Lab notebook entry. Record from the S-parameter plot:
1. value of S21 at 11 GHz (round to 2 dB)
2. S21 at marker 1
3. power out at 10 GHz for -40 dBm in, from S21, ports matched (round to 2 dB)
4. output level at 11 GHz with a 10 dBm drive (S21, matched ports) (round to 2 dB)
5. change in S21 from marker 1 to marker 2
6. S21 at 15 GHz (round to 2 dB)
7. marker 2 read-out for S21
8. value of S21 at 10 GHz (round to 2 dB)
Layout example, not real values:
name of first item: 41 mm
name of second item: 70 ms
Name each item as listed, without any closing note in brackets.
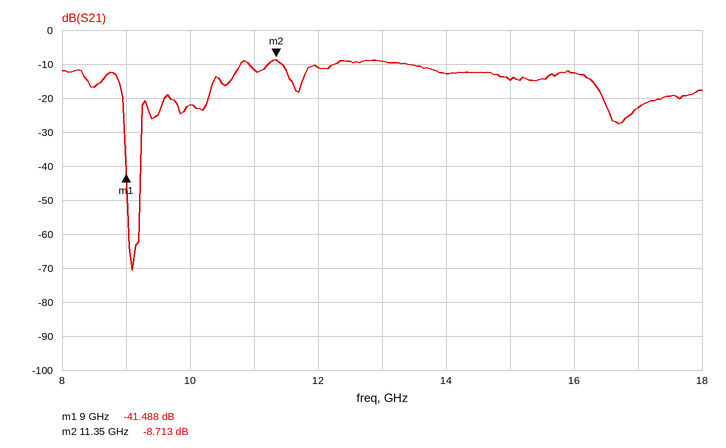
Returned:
value of S21 at 11 GHz: -12 dB
S21 at marker 1: -41.488 dB
power out at 10 GHz for -40 dBm in, from S21, ports matched: -62 dBm
output level at 11 GHz with a 10 dBm drive (S21, matched ports): -2 dBm
change in S21 from marker 1 to marker 2: 32.775 dB
S21 at 15 GHz: -14 dB
marker 2 read-out for S21: -8.713 dB
value of S21 at 10 GHz: -22 dB
